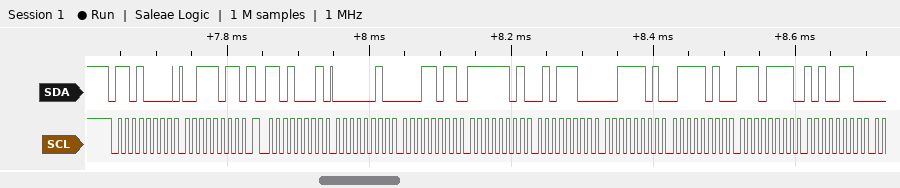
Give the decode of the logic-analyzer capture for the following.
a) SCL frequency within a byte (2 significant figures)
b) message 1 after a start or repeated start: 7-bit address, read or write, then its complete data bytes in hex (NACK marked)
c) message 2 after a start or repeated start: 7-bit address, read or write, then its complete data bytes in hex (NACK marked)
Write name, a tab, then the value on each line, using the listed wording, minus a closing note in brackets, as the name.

SCL frequency within a byte	100 kHz
message 1 after a start or repeated start: 7-bit address, read or write, then its complete data bytes in hex	0x68 write: 3B
message 2 after a start or repeated start: 7-bit address, read or write, then its complete data bytes in hex	0x68 read: 02 1B FD 5C 3D 7A EF A6
